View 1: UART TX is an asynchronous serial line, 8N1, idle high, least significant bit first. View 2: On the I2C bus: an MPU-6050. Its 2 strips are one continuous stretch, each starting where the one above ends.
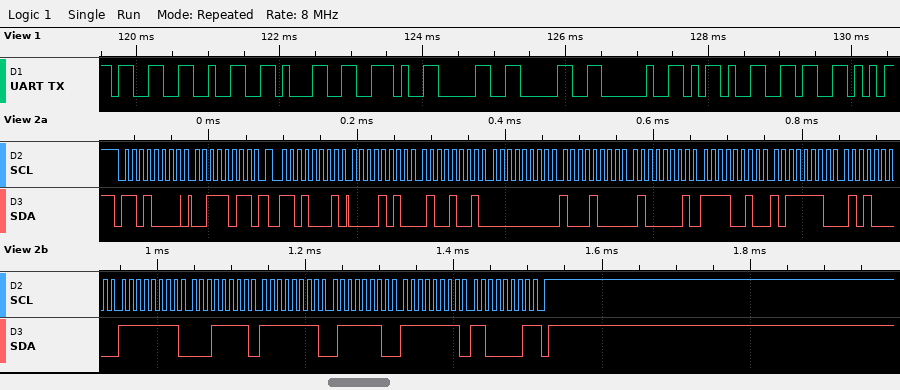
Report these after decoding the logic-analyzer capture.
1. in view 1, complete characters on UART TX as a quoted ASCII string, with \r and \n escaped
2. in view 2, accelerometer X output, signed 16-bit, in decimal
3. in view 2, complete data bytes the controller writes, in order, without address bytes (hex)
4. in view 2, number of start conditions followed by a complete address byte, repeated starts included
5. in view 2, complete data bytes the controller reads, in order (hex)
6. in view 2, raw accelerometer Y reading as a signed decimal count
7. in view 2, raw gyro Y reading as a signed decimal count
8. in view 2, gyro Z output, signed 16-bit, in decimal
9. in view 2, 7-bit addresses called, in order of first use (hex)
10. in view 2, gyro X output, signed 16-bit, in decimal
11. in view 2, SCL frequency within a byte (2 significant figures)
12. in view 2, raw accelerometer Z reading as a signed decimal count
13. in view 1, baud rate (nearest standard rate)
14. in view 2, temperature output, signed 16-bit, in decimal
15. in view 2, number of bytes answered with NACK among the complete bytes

"321.00 -6"
2633
3B
2
0A 49 00 88 41 F2 BE 50 FF 1F FF 7E FF C1
136
-130
-63
0x68
-225
100 kHz
16882
9600 baud
-16816
1
